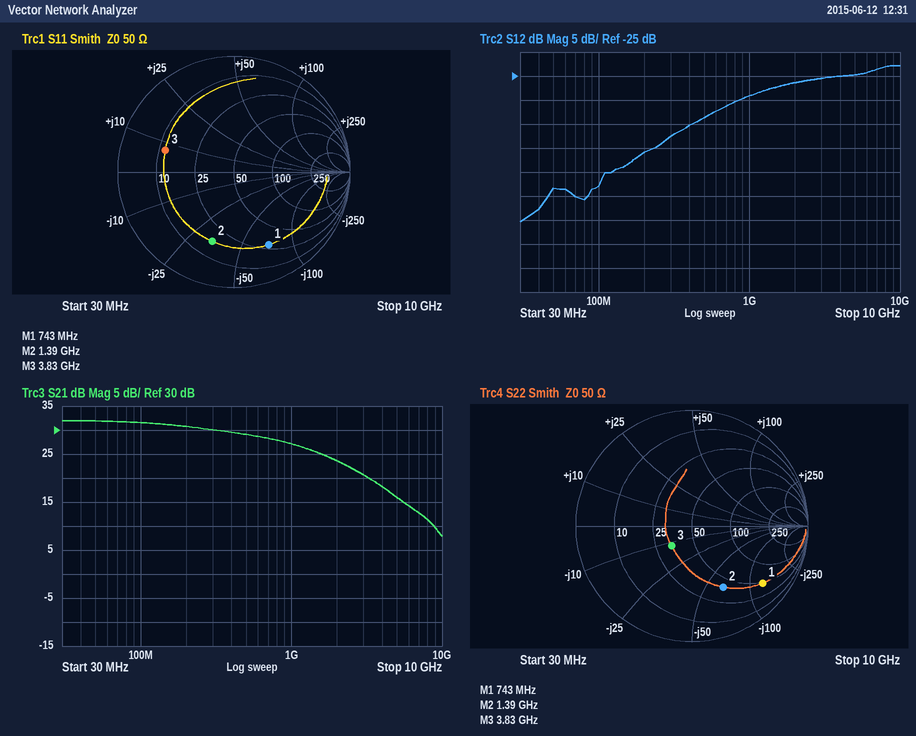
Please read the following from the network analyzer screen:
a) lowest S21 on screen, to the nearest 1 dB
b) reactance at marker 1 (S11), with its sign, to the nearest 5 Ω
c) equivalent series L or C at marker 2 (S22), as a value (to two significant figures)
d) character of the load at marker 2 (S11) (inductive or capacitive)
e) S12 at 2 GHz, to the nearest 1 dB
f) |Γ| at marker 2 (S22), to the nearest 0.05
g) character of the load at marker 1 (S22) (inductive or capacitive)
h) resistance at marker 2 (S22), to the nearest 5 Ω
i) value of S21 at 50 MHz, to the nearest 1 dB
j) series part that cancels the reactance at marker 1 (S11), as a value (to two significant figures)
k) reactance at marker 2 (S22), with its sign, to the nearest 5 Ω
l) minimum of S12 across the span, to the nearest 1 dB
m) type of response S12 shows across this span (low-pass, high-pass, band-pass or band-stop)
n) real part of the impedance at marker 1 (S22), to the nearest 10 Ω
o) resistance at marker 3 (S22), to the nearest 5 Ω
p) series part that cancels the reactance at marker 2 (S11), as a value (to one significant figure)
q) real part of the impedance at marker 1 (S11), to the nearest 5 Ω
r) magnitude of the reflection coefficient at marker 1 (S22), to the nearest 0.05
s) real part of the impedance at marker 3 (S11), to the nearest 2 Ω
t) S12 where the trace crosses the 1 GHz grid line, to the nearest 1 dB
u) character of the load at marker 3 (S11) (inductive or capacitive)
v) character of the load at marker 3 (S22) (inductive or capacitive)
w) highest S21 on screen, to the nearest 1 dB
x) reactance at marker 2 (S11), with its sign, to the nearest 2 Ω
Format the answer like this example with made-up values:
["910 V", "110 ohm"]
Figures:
["8 dB", "-70 Ω", "1.8 pF", "capacitive", "-26 dB", "0.60", "capacitive", "40 Ω", "32 dB", "15 nH", "-65 Ω", "-55 dB", "high-pass", "50 Ω", "35 Ω", "4 nH", "30 Ω", "0.80", "12 Ω", "-29 dB", "inductive", "capacitive", "32 dB", "-34 Ω"]
